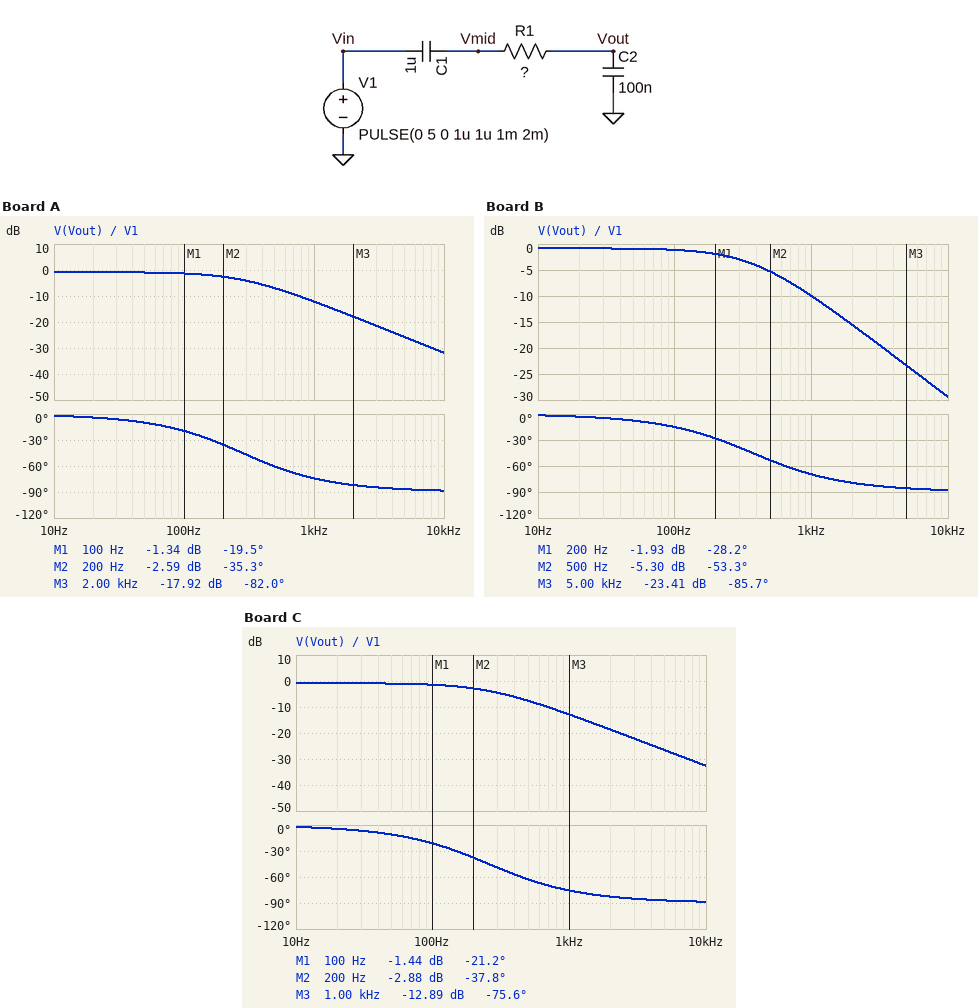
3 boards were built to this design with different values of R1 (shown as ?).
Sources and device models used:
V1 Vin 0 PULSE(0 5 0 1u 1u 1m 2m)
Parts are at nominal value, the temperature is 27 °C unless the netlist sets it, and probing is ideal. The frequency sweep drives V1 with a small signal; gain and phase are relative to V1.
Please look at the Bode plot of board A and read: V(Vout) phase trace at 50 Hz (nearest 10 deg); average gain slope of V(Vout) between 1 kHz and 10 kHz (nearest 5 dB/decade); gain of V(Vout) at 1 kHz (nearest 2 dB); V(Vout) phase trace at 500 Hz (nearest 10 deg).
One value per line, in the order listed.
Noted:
-10 deg
-20 dB/decade
-12 dB
-60 deg
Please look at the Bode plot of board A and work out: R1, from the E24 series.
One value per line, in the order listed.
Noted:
6.2 kΩ
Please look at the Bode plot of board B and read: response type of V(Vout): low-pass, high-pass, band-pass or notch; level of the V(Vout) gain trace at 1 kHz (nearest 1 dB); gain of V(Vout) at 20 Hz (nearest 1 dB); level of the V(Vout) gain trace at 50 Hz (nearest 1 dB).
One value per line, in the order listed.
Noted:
low-pass
-10 dB
-1 dB
-1 dB
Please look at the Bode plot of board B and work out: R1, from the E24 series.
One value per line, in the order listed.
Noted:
4.7 kΩ
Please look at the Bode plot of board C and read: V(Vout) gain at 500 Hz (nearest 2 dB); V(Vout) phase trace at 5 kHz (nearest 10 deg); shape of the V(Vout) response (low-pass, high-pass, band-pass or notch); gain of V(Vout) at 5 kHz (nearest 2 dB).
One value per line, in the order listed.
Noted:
-8 dB
-90 deg
low-pass
-26 dB
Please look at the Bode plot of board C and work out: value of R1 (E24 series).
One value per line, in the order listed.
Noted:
6.8 kΩ
